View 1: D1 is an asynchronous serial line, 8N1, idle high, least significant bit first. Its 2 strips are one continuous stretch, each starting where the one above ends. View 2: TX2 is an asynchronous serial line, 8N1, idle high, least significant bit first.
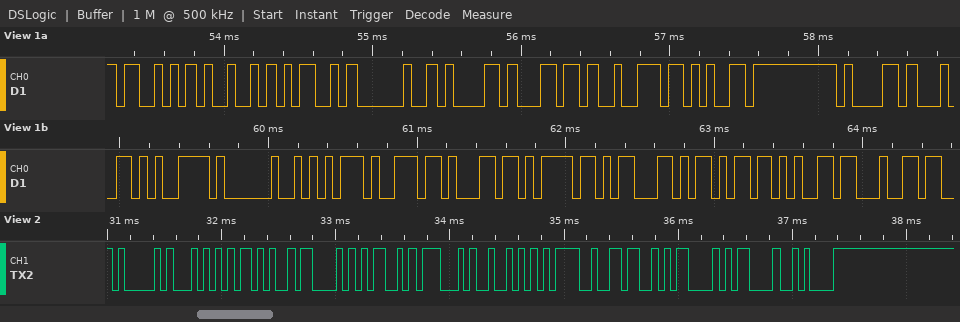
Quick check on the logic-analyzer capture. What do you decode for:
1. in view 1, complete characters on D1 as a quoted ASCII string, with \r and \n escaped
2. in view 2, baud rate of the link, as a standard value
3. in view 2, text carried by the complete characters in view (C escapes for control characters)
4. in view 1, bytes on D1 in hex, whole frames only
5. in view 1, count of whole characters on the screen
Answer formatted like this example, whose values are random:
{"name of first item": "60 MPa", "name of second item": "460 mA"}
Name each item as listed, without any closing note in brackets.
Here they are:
{"in view 1, complete characters on D1 as a quoted ASCII string, with \\r and \\n escaped": "\"SIM already unlocked\"", "in view 2, baud rate of the link, as a standard value": "19200 baud", "in view 2, text carried by the complete characters in view": "\"AT+CMGR=6\\r\\r\\n\"", "in view 1, bytes on D1 in hex, whole frames only": "53 49 4D 20 61 6C 72 65 61 64 79 20 75 6E 6C 6F 63 6B 65 64", "in view 1, count of whole characters on the screen": "20"}
